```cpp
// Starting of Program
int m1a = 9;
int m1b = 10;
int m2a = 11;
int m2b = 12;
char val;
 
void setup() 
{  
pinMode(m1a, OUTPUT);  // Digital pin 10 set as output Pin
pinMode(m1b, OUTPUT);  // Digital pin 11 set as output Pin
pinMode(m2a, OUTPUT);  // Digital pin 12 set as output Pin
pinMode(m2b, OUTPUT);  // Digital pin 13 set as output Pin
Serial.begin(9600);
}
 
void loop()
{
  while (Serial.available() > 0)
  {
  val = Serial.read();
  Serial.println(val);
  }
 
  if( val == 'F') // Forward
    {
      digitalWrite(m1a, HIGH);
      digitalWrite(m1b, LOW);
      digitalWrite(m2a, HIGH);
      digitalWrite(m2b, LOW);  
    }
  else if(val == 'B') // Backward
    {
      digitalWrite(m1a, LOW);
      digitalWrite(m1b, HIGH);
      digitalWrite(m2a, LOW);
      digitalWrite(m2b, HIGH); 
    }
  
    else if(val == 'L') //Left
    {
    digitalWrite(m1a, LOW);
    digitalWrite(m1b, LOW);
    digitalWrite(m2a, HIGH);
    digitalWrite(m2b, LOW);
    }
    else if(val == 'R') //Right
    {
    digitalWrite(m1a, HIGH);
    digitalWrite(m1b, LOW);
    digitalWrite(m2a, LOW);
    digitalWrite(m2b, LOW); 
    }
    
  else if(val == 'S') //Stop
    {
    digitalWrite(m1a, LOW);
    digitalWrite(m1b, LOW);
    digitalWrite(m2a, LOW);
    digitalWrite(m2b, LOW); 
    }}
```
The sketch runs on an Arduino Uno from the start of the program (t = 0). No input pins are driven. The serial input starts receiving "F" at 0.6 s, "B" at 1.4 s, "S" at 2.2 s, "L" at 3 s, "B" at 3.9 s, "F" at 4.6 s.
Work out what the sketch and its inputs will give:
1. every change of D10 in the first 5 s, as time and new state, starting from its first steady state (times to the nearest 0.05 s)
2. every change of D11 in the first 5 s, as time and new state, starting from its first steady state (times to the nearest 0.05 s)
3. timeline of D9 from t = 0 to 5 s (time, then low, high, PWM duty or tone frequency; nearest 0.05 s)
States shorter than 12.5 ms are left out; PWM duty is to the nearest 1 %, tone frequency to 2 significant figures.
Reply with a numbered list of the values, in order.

1. 0 s low; 1.4 s high; 2.2 s low; 3.9 s high; 4.6 s low
2. 0 s low; 0.6 s high; 1.4 s low; 3 s high; 3.9 s low; 4.6 s high
3. 0 s low; 0.6 s high; 1.4 s low; 4.6 s high
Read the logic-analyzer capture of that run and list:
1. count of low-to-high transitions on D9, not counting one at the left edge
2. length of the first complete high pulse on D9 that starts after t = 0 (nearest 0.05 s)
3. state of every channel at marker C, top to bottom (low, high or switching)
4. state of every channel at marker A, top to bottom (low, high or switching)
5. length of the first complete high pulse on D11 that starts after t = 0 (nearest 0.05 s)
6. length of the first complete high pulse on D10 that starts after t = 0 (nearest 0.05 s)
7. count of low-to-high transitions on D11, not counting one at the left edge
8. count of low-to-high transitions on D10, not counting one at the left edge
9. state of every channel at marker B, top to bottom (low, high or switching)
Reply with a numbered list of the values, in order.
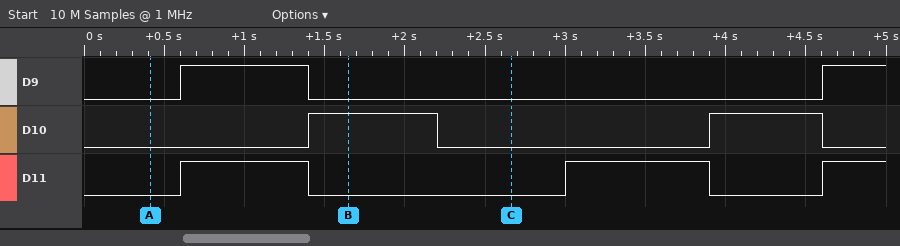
1. 2
2. 0.80 s
3. D9 low, D10 low, D11 low
4. D9 low, D10 low, D11 low
5. 0.80 s
6. 0.80 s
7. 3
8. 2
9. D9 low, D10 high, D11 low
